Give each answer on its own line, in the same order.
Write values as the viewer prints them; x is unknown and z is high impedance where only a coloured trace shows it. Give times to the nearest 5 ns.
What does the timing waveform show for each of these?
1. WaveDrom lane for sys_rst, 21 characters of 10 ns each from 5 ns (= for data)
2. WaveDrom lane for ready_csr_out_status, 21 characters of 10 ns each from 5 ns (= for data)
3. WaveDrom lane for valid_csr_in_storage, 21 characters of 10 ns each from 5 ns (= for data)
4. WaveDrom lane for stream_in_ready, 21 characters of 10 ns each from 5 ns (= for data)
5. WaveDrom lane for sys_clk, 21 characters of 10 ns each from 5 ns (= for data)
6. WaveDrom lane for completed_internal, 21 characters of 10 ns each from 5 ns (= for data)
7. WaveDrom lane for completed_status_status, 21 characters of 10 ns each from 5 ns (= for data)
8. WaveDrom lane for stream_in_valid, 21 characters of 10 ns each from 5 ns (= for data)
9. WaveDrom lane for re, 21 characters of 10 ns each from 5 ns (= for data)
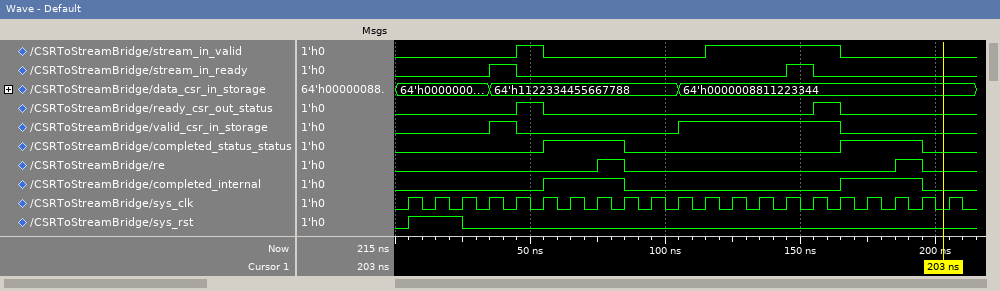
{name: 'sys_rst', wave: '1.0..................'}
{name: 'ready_csr_out_status', wave: '0...10.........10....'}
{name: 'valid_csr_in_storage', wave: '0..10.....1.....0....'}
{name: 'stream_in_ready', wave: '0..10.........10.....'}
{name: 'sys_clk', wave: 'p....................'}
{name: 'completed_internal', wave: '0....1..0.......1..0.'}
{name: 'completed_status_status', wave: '0....1..0.......1..0.'}
{name: 'stream_in_valid', wave: '0...10.....1....0....'}
{name: 're', wave: '0......10.........10.'}
